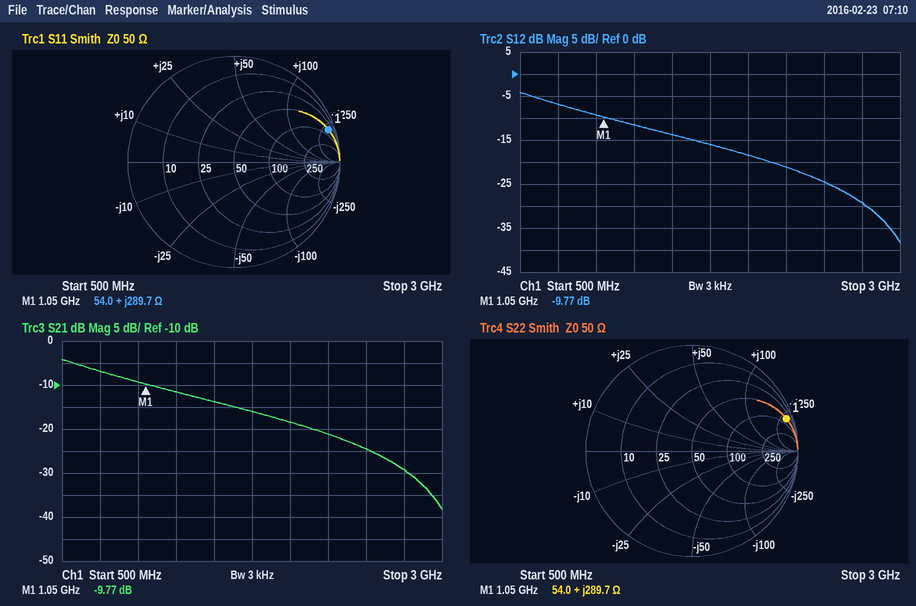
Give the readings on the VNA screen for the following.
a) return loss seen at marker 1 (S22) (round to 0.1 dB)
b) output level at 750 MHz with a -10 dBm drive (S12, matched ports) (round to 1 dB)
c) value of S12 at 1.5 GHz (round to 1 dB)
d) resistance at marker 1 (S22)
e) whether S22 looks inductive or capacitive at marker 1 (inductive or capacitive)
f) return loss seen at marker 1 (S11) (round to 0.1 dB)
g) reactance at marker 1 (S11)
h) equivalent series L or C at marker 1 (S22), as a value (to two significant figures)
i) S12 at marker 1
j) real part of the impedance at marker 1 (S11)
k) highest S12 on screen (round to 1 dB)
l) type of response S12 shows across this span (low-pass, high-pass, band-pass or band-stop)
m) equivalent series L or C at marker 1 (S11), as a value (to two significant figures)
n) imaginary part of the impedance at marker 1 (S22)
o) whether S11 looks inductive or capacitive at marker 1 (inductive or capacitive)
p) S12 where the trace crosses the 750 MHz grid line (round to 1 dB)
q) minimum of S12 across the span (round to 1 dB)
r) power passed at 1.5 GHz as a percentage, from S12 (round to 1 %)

0.5 dB
-17 dBm
-14 dB
54.0 Ω
inductive
0.5 dB
+289.7 Ω
44 nH
-9.77 dB
54.0 Ω
-4 dB
low-pass
44 nH
+289.7 Ω
inductive
-7 dB
-38 dB
4 %
